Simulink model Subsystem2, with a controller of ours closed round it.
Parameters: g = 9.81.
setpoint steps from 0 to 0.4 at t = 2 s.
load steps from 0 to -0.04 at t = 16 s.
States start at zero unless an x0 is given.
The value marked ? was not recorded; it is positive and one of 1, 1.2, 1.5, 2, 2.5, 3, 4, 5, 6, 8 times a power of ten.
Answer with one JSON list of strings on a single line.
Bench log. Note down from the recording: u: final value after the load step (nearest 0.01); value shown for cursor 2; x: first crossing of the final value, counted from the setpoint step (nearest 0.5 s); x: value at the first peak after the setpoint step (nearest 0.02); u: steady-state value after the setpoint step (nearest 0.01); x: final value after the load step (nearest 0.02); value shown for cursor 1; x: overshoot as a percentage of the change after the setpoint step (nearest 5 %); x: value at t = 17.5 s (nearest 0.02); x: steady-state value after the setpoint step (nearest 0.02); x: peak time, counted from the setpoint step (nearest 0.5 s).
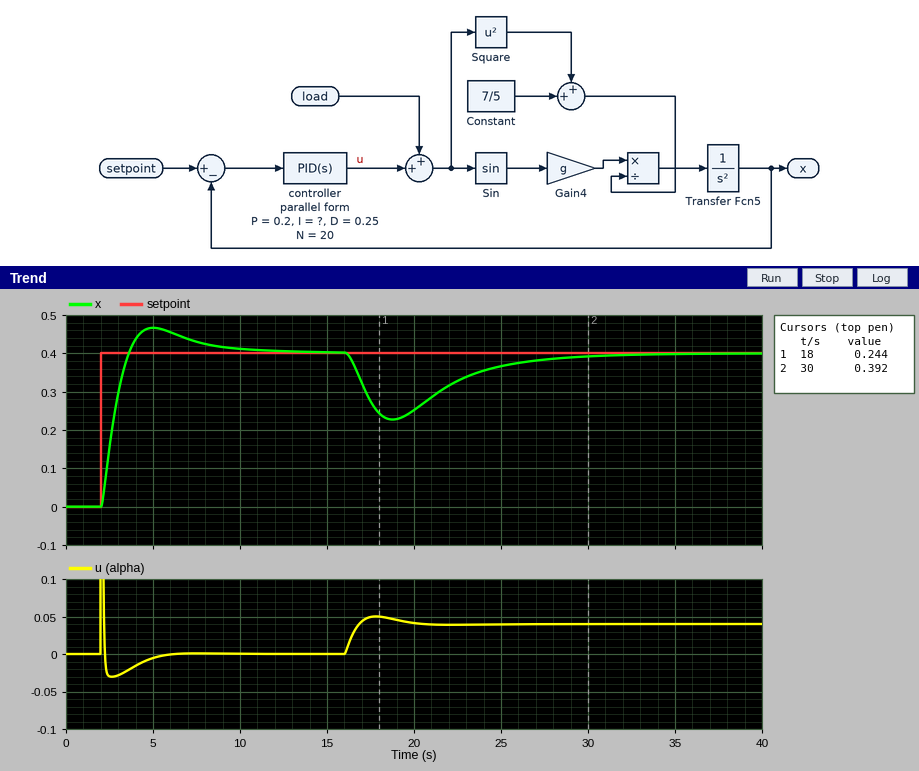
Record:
["0.04", "0.392", "1.5 s", "0.46", "0.00", "0.40", "0.244", "15 %", "0.28", "0.40", "3.0 s"]
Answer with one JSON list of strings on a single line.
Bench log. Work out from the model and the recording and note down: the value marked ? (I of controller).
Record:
["0.04"]
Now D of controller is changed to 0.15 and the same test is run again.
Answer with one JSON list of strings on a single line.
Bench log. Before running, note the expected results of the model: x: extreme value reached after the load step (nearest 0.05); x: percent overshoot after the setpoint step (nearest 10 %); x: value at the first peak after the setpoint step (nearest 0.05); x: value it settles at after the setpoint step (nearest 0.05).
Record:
["0.20", "40 %", "0.55", "0.40"]
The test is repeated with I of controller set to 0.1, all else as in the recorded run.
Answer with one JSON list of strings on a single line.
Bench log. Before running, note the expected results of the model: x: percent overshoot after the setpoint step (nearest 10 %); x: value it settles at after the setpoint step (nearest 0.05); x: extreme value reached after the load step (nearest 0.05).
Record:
["30 %", "0.40", "0.25"]
